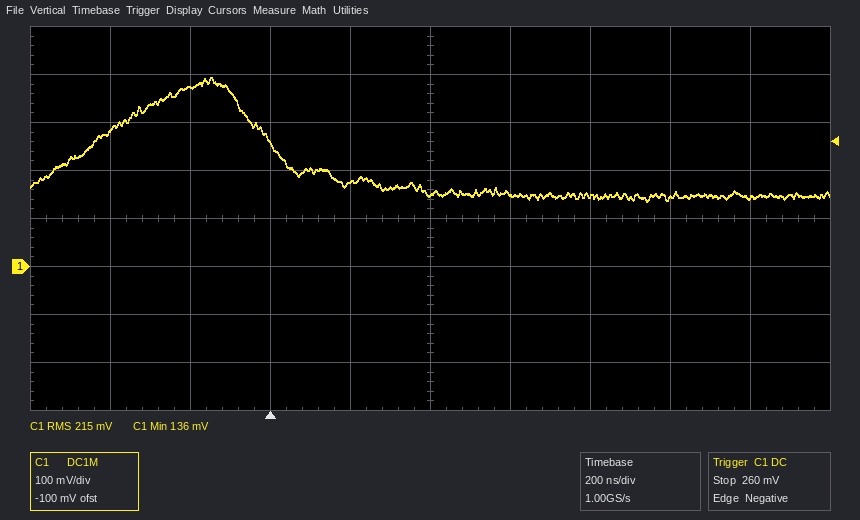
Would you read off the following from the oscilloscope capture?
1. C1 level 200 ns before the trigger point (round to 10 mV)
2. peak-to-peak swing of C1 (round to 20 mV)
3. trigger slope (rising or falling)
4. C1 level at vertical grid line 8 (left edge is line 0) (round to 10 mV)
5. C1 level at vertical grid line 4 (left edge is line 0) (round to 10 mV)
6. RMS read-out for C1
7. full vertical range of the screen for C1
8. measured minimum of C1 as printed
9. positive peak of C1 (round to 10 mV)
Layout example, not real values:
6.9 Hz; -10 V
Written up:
370 mV; 260 mV; falling; 140 mV; 170 mV; 215 mV; 800 mV; 136 mV; 390 mV
